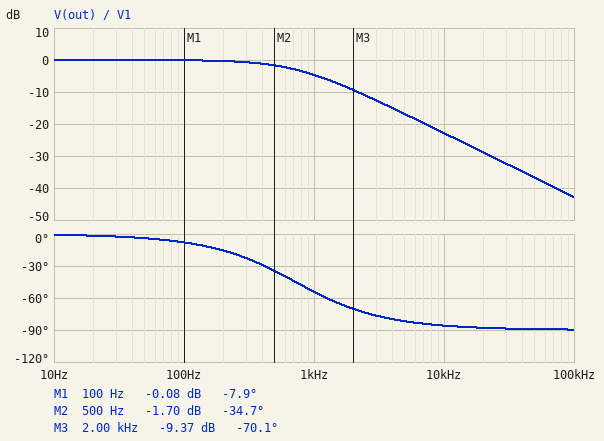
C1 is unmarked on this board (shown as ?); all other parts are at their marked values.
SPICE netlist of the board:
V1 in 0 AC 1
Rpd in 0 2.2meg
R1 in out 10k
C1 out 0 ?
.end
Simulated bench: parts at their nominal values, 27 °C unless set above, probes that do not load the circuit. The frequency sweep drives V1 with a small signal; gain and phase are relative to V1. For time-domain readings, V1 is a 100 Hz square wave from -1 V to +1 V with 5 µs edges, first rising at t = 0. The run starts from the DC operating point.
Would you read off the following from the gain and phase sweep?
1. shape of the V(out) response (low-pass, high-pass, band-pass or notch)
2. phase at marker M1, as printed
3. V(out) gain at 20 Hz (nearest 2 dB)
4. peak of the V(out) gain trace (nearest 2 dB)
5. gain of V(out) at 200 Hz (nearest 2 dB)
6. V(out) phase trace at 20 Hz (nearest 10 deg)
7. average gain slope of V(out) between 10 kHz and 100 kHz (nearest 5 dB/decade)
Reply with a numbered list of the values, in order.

1. low-pass
2. -7.9 deg
3. 0 dB
4. 0 dB
5. 0 dB
6. 0 deg
7. -20 dB/decade
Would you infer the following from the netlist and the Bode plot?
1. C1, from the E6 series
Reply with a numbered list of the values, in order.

1. 22 nF
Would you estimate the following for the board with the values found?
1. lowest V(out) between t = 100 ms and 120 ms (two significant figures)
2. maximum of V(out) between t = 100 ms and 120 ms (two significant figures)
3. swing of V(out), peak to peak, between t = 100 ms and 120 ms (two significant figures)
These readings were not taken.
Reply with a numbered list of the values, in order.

1. -1.0 V
2. 1.0 V
3. 2.0 V
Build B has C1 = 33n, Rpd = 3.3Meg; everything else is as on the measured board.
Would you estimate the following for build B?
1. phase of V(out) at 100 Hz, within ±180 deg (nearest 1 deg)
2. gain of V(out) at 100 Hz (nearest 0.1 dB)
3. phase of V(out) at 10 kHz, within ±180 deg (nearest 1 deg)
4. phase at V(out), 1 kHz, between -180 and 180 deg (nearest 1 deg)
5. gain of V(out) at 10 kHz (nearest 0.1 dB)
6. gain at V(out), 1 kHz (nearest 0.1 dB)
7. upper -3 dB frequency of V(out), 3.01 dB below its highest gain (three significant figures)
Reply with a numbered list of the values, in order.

1. -12 deg
2. -0.2 dB
3. -87 deg
4. -64 deg
5. -26.3 dB
6. -7.2 dB
7. 482 Hz
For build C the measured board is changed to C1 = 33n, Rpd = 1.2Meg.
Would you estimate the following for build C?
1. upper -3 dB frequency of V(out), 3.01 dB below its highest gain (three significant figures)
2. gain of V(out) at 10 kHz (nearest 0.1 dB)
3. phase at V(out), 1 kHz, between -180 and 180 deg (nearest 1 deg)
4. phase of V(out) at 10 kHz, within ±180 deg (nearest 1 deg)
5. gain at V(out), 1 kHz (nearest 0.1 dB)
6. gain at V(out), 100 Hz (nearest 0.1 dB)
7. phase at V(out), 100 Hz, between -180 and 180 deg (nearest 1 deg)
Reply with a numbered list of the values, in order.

1. 482 Hz
2. -26.3 dB
3. -64 deg
4. -87 deg
5. -7.2 dB
6. -0.2 dB
7. -12 deg
